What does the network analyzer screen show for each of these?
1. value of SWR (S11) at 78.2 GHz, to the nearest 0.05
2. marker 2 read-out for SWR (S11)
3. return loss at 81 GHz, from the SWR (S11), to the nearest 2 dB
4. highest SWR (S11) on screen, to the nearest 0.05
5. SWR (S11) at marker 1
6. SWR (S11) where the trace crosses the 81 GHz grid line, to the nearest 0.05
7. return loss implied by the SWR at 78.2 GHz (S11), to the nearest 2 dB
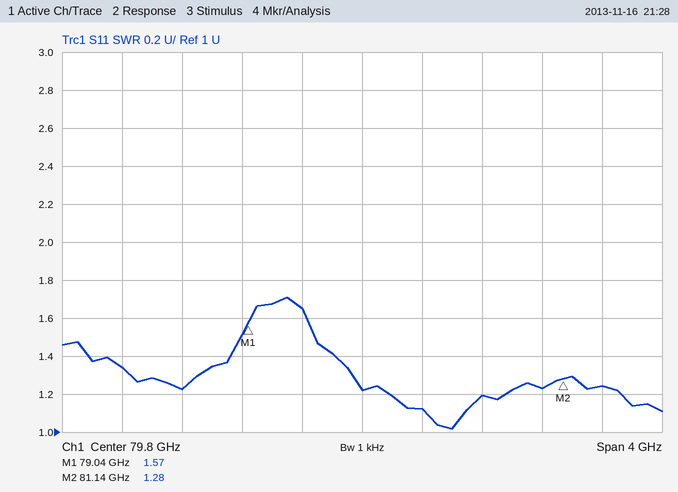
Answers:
1.35
1.28
20 dB
1.70
1.57
1.25
16 dB
